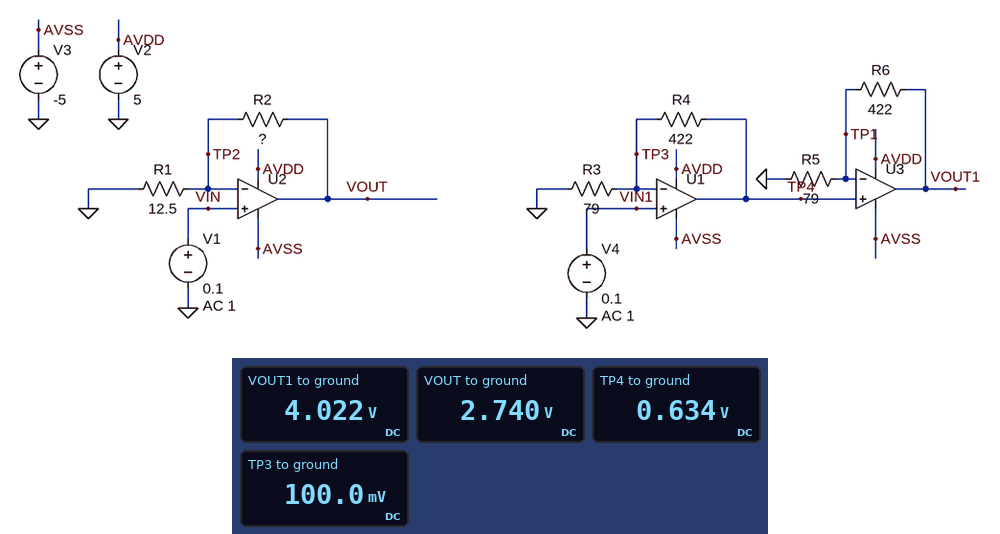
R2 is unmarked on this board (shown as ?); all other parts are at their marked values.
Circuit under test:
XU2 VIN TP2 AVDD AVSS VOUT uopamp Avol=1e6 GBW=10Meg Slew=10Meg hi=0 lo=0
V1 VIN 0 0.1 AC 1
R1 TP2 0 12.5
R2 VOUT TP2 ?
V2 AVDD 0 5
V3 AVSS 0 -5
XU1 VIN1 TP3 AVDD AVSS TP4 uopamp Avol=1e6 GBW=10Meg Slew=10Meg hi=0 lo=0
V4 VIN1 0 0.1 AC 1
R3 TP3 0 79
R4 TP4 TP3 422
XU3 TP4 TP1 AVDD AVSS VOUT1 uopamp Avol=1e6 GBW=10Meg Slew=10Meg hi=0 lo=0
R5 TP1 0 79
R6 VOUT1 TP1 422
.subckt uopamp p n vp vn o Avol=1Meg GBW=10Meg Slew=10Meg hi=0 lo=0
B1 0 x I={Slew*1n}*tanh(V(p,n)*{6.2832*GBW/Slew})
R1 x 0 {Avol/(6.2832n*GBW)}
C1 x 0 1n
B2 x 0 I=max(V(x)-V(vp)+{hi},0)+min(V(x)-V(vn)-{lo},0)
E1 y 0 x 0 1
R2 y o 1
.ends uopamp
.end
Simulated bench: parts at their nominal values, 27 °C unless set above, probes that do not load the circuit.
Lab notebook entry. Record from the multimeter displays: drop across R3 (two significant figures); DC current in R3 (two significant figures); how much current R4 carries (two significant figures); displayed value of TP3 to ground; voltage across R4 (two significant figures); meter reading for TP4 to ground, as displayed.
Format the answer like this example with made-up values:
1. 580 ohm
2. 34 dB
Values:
1. 100 mV
2. 1.3 mA
3. 1.3 mA
4. 100.0 mV
5. 530 mV
6. 0.634 V
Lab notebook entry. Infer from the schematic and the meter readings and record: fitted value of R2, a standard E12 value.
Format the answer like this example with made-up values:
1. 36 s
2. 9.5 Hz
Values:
1. 330 Ω
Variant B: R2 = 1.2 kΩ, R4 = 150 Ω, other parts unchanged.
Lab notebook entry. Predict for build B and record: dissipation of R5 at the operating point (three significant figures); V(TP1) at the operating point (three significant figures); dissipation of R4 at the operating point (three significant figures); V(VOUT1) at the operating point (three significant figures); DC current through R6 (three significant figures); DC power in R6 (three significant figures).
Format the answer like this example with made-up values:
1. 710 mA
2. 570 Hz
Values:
1. 1.06 mW
2. 290 mV
3. 240 µW
4. 1.84 V
5. 3.67 mA
6. 5.68 mW
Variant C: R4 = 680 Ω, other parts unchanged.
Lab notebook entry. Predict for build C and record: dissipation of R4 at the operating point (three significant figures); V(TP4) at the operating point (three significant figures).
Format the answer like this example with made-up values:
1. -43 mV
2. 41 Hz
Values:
1. 1.09 mW
2. 961 mV
